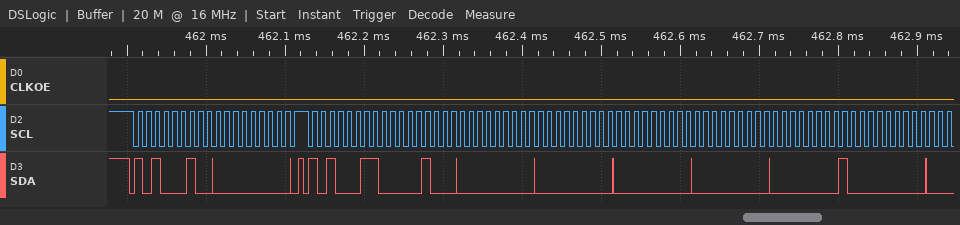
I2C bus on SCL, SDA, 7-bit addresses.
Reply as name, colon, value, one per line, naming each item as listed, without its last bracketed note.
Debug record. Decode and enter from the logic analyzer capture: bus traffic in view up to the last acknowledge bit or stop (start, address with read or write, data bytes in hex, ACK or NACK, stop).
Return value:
bus traffic in view up to the last acknowledge bit or stop: start, address 51 write ACK, 00 ACK, stop, start, address 51 read ACK, 08 ACK, 00 ACK, 00 ACK, 00 ACK, 00 ACK, 01 ACK, 00 ACK
